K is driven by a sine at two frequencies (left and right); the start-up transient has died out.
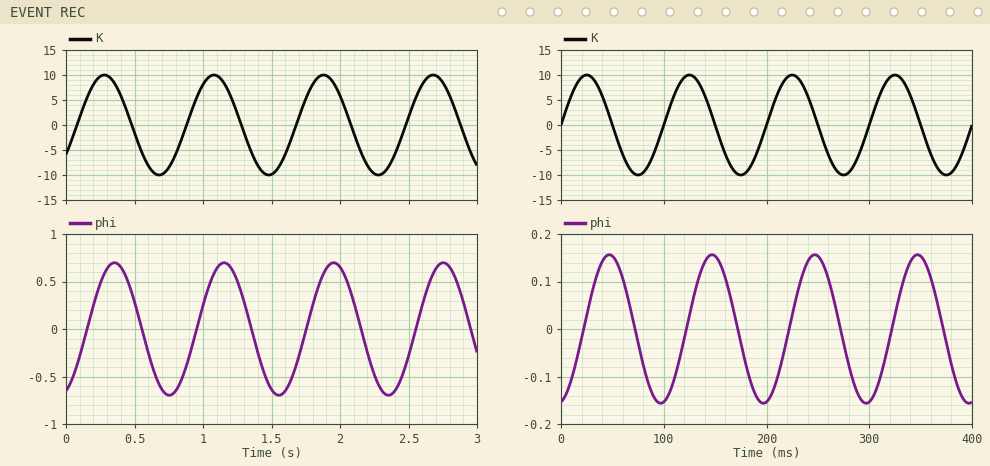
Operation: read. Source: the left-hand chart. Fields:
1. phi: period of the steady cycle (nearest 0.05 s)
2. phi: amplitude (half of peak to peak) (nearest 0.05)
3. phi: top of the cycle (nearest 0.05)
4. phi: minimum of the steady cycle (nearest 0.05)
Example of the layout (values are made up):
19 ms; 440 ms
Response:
0.80 s; 0.70; 0.70; -0.70
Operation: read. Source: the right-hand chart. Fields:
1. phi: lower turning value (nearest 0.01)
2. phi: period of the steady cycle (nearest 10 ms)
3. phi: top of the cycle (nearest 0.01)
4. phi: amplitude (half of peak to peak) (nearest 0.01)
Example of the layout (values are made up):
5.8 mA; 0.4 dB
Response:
-0.16; 100 ms; 0.16; 0.16
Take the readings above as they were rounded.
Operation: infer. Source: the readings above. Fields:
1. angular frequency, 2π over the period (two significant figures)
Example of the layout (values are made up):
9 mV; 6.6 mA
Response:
0.063 rad/ms
